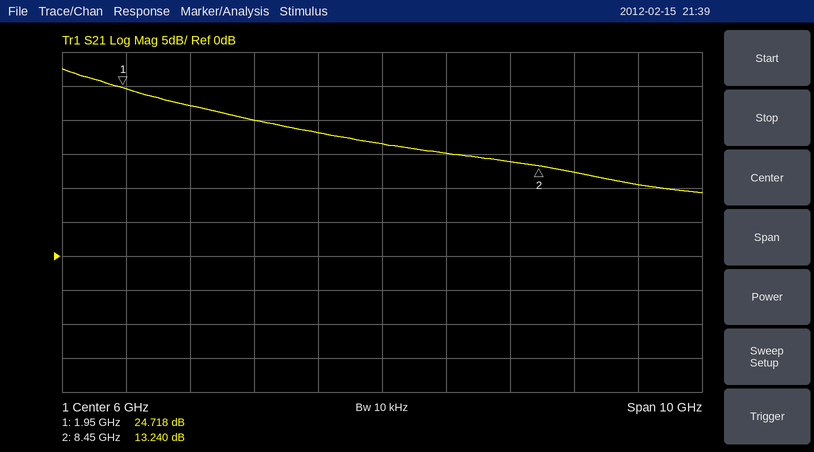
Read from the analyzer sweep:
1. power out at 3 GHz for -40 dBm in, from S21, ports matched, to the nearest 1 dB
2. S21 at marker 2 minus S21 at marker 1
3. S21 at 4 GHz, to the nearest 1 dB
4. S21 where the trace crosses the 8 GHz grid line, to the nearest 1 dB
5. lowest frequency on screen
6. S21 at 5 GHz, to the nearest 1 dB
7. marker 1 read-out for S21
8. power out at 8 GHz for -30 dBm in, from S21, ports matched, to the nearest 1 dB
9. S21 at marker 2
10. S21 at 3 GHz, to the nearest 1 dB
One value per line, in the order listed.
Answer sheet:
-18 dBm
-11.478 dB
20 dB
14 dB
1 GHz
18 dB
24.718 dB
-16 dBm
13.240 dB
22 dB
